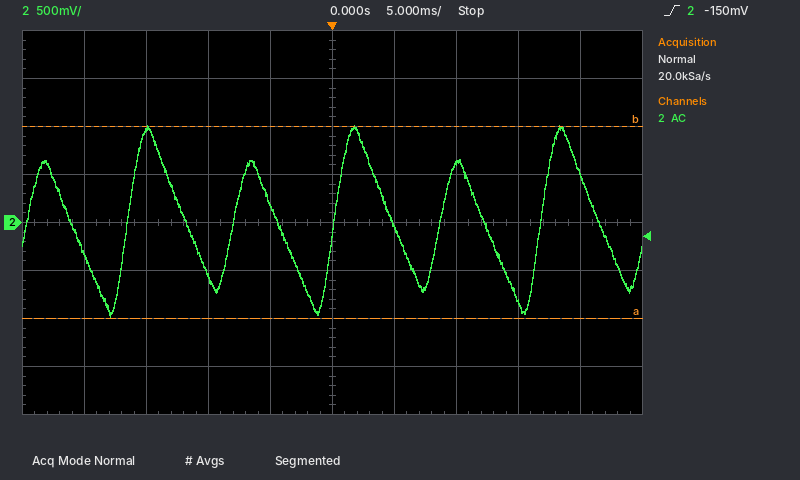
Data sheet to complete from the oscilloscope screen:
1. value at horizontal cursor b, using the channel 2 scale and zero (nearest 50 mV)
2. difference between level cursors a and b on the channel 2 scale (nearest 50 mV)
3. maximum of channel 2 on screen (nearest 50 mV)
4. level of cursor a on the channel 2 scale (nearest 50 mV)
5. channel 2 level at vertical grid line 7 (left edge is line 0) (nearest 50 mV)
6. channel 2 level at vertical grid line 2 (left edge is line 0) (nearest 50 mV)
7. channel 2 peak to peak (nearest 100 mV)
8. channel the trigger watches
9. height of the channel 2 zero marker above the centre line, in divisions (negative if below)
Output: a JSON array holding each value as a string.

["1.00 V", "2.00 V", "1.00 V", "-1.00 V", "600 mV", "950 mV", "2.00 V", "channel 2", "0.0 div"]
